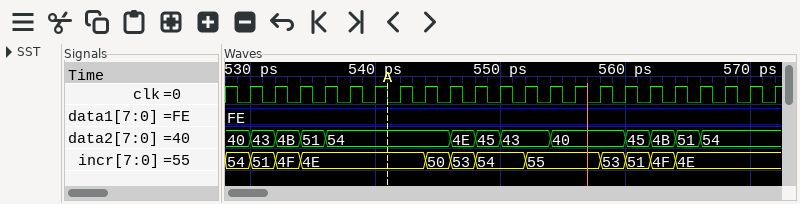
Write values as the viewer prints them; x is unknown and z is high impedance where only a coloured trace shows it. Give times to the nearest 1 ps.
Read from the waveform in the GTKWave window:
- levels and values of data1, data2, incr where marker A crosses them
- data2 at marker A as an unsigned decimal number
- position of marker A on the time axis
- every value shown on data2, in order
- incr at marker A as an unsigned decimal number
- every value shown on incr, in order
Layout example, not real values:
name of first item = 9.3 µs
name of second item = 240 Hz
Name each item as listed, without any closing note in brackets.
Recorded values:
levels and values of data1, data2, incr where marker A crosses them = data1=FE, data2=54, incr=4E
data2 at marker A as an unsigned decimal number = 84
position of marker A on the time axis = 541 ps
every value shown on data2, in order = 40, 43, 4B, 51, 54, 4E, 45, 43, 40, 45, 4B, 51, 54
incr at marker A as an unsigned decimal number = 78
every value shown on incr, in order = 54, 51, 4F, 4E, 50, 53, 54, 55, 53, 51, 4F, 4E
